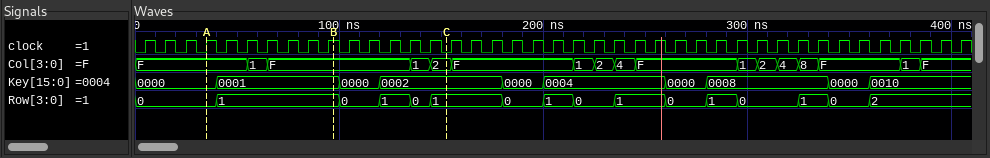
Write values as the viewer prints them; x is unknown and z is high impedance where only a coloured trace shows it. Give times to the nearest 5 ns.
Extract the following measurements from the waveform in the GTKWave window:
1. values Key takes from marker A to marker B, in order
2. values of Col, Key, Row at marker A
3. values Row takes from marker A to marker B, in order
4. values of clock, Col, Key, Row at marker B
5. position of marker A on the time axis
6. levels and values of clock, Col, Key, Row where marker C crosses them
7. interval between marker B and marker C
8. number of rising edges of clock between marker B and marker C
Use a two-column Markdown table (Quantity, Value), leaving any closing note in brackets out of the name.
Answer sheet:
| Quantity | Value |
|---|---|
| values Key takes from marker A to marker B, in order | 0000, 0001 |
| values of Col, Key, Row at marker A | Col=F, Key=0000, Row=0 |
| values Row takes from marker A to marker B, in order | 0, 1 |
| values of clock, Col, Key, Row at marker B | clock=1, Col=F, Key=0001, Row=1 |
| position of marker A on the time axis | 35 ns |
| levels and values of clock, Col, Key, Row where marker C crosses them | clock=0, Col=2, Key=0002, Row=1 |
| interval between marker B and marker C | 55 ns |
| number of rising edges of clock between marker B and marker C | 5 |
